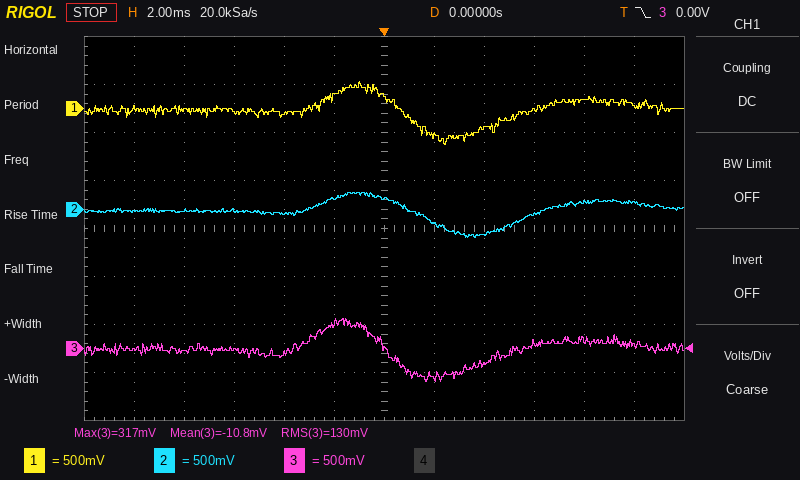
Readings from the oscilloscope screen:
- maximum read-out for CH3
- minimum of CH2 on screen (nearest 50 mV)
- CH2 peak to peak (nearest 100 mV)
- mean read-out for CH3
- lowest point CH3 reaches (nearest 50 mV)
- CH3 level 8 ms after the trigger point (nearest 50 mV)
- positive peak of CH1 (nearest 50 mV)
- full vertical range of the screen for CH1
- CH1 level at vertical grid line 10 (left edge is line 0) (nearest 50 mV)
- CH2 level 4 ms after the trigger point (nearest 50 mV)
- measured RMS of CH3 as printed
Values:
317 mV
-300 mV
500 mV
-10.8 mV
-350 mV
100 mV
300 mV
4 V
100 mV
-250 mV
130 mV
